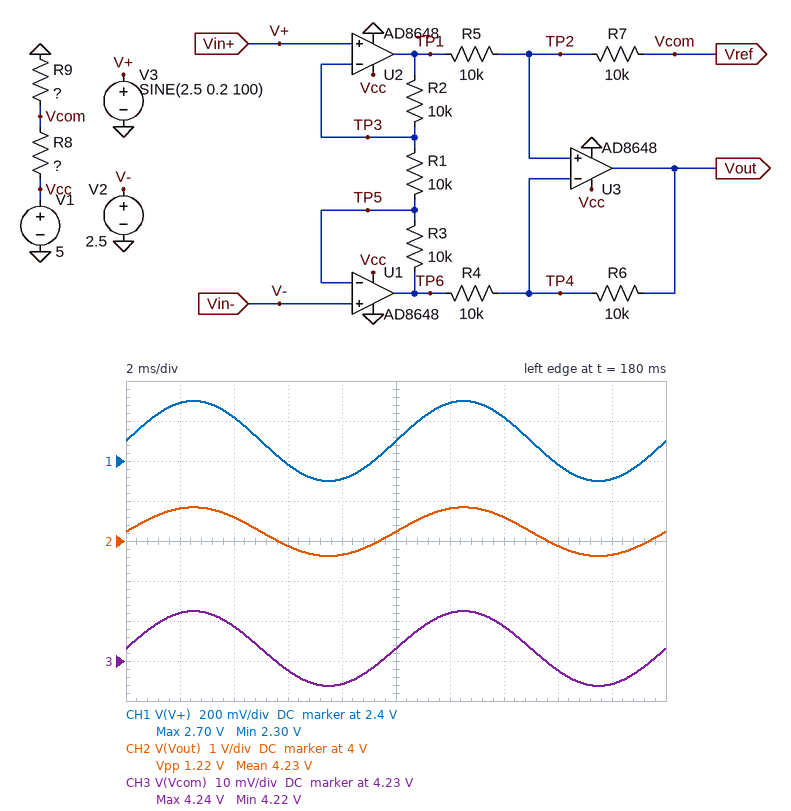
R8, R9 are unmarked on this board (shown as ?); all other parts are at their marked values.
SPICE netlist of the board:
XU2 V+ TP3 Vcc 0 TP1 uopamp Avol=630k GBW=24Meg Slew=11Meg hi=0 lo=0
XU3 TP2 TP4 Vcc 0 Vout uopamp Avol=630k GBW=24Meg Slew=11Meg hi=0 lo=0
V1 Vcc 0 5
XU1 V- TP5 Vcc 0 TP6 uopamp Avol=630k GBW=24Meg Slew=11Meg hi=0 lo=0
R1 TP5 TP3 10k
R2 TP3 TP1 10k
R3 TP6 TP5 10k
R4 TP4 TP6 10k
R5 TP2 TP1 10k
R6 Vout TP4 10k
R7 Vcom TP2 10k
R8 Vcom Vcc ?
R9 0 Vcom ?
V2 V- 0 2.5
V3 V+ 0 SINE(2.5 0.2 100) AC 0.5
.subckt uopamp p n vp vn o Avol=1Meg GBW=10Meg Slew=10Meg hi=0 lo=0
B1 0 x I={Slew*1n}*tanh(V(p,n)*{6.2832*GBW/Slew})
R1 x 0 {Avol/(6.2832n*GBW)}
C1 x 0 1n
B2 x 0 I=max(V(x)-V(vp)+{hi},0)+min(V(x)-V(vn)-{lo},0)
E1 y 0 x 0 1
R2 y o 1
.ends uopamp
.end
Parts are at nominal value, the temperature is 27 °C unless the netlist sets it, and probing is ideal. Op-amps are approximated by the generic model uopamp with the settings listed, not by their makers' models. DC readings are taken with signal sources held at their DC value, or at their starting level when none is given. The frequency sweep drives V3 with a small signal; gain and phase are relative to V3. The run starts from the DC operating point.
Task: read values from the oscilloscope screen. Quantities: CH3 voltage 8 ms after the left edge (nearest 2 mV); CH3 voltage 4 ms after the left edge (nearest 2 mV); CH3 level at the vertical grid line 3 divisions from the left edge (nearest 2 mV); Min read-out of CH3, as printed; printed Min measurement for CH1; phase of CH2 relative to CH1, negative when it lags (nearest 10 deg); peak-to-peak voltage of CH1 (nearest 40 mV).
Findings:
4.224 V
4.238 V
4.228 V
4.22 V
2.30 V
0 deg
400 mV
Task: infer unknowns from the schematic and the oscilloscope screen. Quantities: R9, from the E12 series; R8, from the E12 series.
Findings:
3.3 kΩ
560 Ω
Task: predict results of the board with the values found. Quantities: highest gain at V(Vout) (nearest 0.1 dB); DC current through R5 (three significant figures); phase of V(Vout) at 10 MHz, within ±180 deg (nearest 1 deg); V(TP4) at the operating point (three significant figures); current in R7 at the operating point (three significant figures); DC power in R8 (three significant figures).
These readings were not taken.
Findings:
9.7 dB
86.7 µA
-91 deg
3.37 V
86.7 µA
1.05 mW
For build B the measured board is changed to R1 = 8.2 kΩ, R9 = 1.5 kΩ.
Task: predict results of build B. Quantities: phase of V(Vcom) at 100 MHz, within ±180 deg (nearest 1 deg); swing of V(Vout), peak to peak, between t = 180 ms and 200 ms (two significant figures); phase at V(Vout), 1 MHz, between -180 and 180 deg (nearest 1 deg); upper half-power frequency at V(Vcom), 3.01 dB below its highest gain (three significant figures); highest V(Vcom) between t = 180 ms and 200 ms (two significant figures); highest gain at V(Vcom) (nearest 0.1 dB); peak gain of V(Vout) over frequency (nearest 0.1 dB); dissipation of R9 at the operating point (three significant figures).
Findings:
-81 deg
1.4 V
-13 deg
7.87 MHz
3.6 V
-27.1 dB
10.8 dB
8.73 mW
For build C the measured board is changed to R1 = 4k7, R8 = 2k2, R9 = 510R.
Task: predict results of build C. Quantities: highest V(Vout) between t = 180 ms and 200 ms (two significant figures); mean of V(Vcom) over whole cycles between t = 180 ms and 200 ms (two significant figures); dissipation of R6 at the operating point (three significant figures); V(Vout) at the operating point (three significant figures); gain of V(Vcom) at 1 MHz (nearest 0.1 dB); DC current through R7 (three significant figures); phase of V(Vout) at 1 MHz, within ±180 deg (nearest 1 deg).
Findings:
2.0 V
970 mV
58.3 µW
973 mV
-24.1 dB
76.4 µA
-17 deg
